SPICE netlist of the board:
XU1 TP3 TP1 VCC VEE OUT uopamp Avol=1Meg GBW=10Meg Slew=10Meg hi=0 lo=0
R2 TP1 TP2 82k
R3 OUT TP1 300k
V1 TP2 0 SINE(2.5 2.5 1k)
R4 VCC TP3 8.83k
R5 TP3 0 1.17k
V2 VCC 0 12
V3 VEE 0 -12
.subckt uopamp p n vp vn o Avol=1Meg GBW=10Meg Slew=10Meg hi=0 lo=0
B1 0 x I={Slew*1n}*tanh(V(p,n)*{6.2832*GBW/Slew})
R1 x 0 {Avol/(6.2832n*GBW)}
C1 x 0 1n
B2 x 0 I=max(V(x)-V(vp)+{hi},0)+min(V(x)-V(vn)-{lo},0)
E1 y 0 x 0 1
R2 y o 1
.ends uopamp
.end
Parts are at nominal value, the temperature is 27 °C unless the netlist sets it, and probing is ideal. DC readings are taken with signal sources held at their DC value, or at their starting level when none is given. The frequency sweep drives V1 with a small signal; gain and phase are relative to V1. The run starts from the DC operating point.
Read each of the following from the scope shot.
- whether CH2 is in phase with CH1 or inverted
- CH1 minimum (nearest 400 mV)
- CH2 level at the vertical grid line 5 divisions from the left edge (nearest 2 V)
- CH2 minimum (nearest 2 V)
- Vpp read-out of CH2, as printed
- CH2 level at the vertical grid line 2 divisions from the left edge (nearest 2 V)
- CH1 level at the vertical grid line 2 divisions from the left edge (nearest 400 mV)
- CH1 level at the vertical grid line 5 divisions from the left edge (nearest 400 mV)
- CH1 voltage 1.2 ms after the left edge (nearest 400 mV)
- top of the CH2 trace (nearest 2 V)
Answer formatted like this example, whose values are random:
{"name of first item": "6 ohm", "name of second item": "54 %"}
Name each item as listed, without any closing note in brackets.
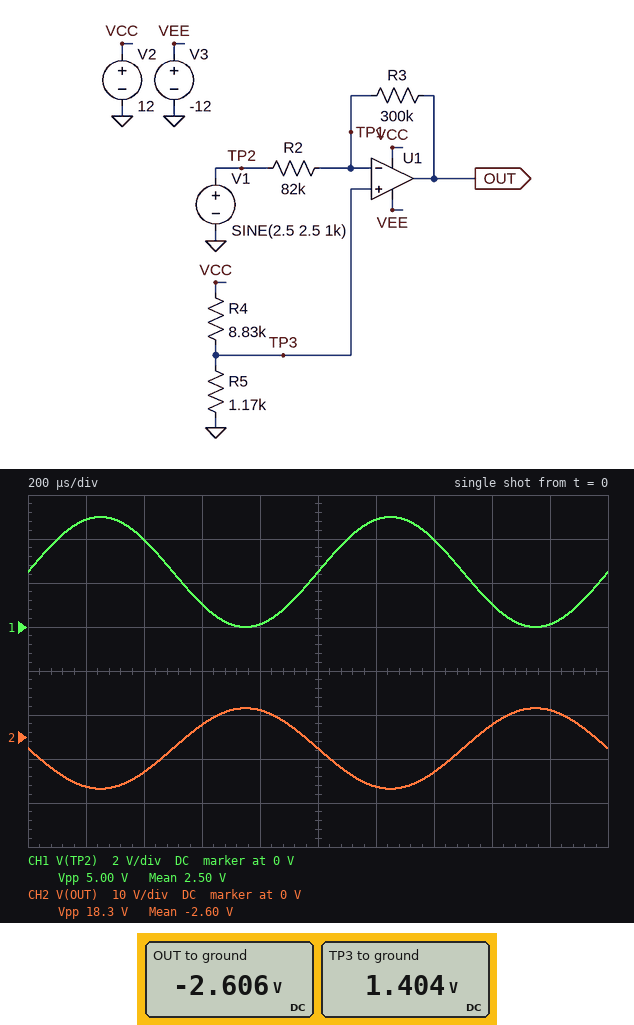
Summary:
{"whether CH2 is in phase with CH1 or inverted": "inverted", "CH1 minimum": "0 V", "CH2 level at the vertical grid line 5 divisions from the left edge": "-2 V", "CH2 minimum": "-12 V", "Vpp read-out of CH2, as printed": "18.3 V", "CH2 level at the vertical grid line 2 divisions from the left edge": "-8 V", "CH1 level at the vertical grid line 2 divisions from the left edge": "4.0 V", "CH1 level at the vertical grid line 5 divisions from the left edge": "2.4 V", "CH1 voltage 1.2 ms after the left edge": "4.8 V", "top of the CH2 trace": "6 V"}
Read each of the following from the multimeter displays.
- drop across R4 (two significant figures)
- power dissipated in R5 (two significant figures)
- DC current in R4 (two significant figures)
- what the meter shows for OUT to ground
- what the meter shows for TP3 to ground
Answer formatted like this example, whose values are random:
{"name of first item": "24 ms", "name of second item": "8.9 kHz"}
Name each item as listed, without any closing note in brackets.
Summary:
{"drop across R4": "11 V", "power dissipated in R5": "1.7 mW", "DC current in R4": "1.2 mA", "what the meter shows for OUT to ground": "-2.606 V", "what the meter shows for TP3 to ground": "1.404 V"}
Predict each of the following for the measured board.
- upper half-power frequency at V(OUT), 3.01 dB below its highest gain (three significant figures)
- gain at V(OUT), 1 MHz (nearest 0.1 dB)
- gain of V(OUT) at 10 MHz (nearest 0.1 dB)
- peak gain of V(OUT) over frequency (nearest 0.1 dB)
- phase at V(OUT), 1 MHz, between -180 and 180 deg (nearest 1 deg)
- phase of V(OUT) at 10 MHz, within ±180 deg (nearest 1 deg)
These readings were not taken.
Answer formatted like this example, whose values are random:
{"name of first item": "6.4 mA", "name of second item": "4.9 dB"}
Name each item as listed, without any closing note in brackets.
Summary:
{"upper half-power frequency at V(OUT), 3.01 dB below its highest gain": "2.15 MHz", "gain at V(OUT), 1 MHz": "10.4 dB", "gain of V(OUT) at 10 MHz": "-2.3 dB", "peak gain of V(OUT) over frequency": "11.3 dB", "phase at V(OUT), 1 MHz, between -180 and 180 deg": "155 deg", "phase of V(OUT) at 10 MHz, within ±180 deg": "102 deg"}
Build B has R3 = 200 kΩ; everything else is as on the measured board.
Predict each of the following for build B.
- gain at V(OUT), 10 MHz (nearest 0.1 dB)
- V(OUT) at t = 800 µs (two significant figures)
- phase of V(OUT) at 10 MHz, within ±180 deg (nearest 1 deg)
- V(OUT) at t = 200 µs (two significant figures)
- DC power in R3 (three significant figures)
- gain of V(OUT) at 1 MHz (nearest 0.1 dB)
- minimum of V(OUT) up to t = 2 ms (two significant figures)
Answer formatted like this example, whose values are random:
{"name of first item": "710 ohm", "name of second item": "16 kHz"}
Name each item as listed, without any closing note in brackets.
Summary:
{"gain at V(OUT), 10 MHz": "-3.3 dB", "V(OUT) at t = 800 µs": "4.5 V", "phase of V(OUT) at 10 MHz, within ±180 deg": "106 deg", "V(OUT) at t = 200 µs": "-7.1 V", "DC power in R3": "35.7 µW", "gain of V(OUT) at 1 MHz": "7.3 dB", "minimum of V(OUT) up to t = 2 ms": "-7.4 V"}
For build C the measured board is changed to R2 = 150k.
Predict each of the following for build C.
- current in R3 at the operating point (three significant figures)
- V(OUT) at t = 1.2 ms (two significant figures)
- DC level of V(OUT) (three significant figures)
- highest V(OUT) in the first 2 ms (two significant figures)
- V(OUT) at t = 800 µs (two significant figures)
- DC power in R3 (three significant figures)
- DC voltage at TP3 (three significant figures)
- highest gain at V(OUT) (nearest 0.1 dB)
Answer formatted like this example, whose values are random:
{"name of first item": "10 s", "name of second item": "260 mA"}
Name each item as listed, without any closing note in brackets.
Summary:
{"current in R3 at the operating point": "7.31 µA", "V(OUT) at t = 1.2 ms": "-5.5 V", "DC level of V(OUT)": "-788 mV", "highest V(OUT) in the first 2 ms": "4.2 V", "V(OUT) at t = 800 µs": "4.0 V", "DC power in R3": "16.0 µW", "DC voltage at TP3": "1.40 V", "highest gain at V(OUT)": "6.0 dB"}
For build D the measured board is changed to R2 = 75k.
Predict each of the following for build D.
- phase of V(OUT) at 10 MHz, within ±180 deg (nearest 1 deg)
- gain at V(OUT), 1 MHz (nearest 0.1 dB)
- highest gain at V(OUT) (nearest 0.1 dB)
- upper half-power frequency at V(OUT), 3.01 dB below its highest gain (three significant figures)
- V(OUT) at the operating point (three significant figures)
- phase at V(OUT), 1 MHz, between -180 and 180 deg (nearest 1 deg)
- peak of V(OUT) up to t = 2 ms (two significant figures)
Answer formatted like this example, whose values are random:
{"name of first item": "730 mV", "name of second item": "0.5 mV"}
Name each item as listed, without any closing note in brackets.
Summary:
{"phase of V(OUT) at 10 MHz, within ±180 deg": "101 deg", "gain at V(OUT), 1 MHz": "11.1 dB", "highest gain at V(OUT)": "12.0 dB", "upper half-power frequency at V(OUT), 3.01 dB below its highest gain": "2.00 MHz", "V(OUT) at the operating point": "-2.98 V", "phase at V(OUT), 1 MHz, between -180 and 180 deg": "153 deg", "peak of V(OUT) up to t = 2 ms": "7.0 V"}
